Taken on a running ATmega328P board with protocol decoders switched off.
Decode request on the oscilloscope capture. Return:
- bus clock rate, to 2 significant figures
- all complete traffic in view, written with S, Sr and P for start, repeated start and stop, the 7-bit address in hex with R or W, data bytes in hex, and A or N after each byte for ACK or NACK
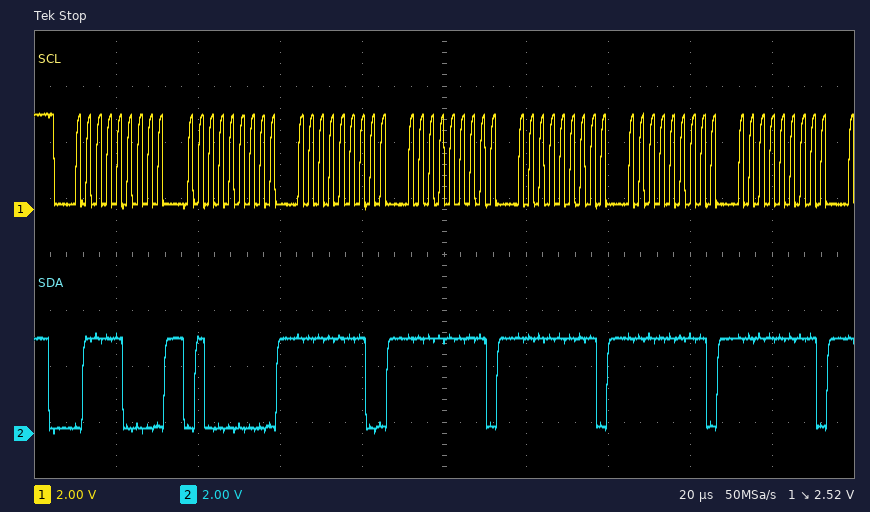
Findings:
400 kHz
S 3CW A 40 A FE A FF A FF A FF A FF A
